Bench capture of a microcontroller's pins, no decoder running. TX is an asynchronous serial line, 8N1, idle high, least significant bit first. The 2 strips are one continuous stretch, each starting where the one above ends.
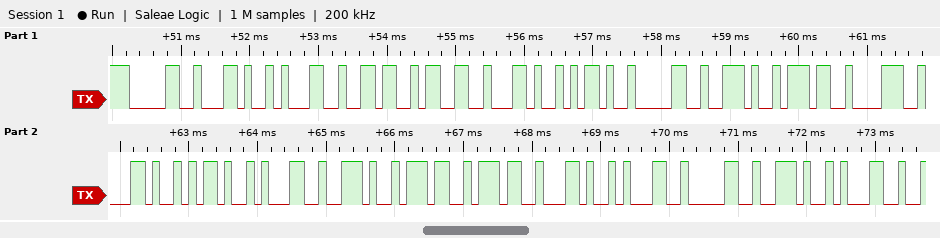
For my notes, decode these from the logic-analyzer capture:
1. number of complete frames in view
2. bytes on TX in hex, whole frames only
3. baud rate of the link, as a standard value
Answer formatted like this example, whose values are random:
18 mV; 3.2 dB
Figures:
22; 30 2C 31 36 33 2C 2D 30 2E 37 38 2C 2D 31 2E 37 37 2C 31 30 2E 31; 9600 baud
